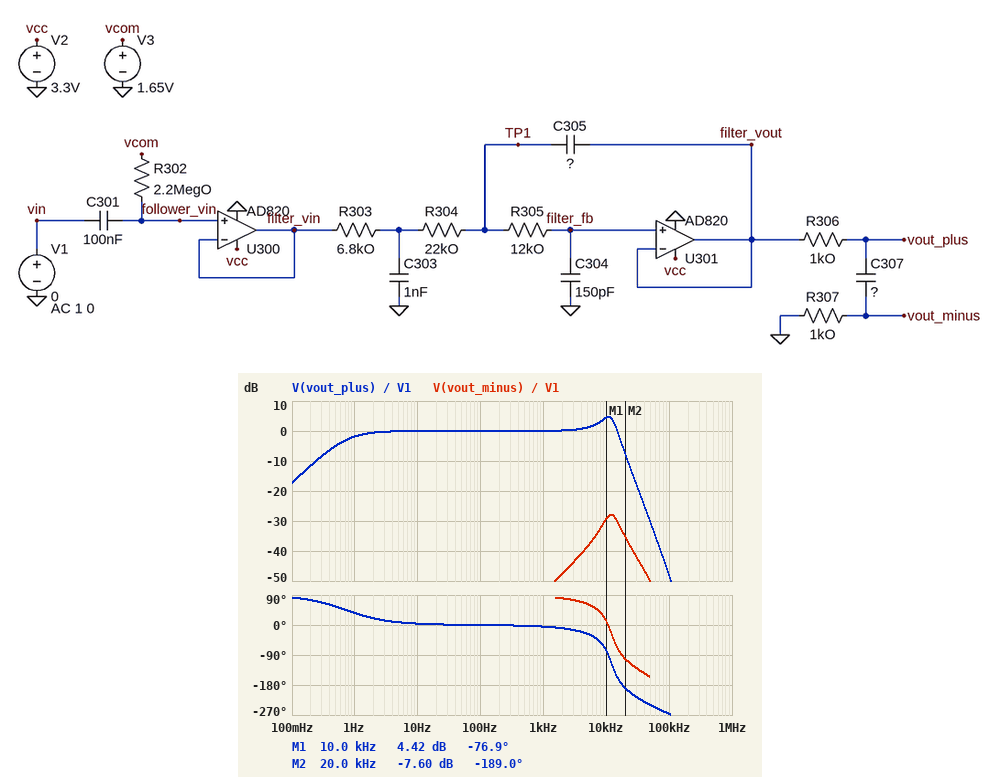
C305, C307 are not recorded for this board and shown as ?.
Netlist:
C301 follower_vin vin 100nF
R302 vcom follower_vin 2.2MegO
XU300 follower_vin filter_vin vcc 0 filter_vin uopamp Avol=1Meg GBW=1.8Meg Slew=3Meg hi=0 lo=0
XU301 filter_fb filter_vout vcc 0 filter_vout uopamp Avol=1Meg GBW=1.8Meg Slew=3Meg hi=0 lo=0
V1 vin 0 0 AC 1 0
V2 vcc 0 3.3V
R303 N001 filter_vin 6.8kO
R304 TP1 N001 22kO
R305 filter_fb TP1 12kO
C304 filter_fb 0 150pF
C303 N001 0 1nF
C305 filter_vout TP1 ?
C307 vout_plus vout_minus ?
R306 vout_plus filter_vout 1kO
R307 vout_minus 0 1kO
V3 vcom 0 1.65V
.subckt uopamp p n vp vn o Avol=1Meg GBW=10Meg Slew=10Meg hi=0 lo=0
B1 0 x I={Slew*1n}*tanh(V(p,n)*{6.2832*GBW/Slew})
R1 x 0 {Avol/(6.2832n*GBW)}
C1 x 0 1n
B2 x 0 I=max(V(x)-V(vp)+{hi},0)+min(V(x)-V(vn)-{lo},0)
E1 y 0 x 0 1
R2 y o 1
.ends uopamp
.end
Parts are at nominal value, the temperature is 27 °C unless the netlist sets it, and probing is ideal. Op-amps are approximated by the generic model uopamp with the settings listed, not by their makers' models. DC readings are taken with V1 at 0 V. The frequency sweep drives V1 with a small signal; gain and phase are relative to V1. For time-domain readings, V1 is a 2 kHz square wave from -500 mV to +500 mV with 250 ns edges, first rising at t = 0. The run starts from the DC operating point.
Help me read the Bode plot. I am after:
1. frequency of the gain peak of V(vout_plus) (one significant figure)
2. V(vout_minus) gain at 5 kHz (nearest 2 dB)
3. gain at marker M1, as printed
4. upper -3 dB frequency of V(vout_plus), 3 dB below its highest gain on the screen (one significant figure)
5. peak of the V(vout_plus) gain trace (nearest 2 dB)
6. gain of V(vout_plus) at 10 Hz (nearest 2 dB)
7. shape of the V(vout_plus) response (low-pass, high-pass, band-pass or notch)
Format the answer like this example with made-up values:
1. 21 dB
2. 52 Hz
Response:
1. 10 kHz
2. -38 dB
3. 4.42 dB
4. 10 kHz
5. 4 dB
6. 0 dB
7. band-pass
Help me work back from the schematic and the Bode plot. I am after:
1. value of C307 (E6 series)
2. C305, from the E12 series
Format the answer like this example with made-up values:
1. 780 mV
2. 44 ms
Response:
1. 330 pF
2. 3.3 nF
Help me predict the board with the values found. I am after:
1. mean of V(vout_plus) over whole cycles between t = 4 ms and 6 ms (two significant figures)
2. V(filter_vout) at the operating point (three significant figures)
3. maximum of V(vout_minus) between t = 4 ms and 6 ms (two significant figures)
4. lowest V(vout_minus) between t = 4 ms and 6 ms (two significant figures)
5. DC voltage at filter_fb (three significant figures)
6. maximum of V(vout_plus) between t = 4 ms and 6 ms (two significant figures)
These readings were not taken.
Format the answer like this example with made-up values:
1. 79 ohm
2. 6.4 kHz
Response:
1. 2.1 V
2. 1.65 V
3. 16 mV
4. -16 mV
5. 1.65 V
6. 3.0 V
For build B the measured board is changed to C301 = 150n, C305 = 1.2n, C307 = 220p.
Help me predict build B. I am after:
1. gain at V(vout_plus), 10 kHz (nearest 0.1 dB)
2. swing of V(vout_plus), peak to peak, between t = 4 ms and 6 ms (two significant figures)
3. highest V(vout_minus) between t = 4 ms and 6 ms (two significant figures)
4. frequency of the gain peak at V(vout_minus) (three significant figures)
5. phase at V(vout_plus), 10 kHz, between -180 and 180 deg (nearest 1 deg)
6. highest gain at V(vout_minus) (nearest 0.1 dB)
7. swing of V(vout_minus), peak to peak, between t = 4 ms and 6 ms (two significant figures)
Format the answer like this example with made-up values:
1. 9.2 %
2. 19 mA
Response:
1. 0.5 dB
2. 1.3 V
3. 13 mV
4. 19.3 kHz
5. -52 deg
6. -32.1 dB
7. 26 mV
